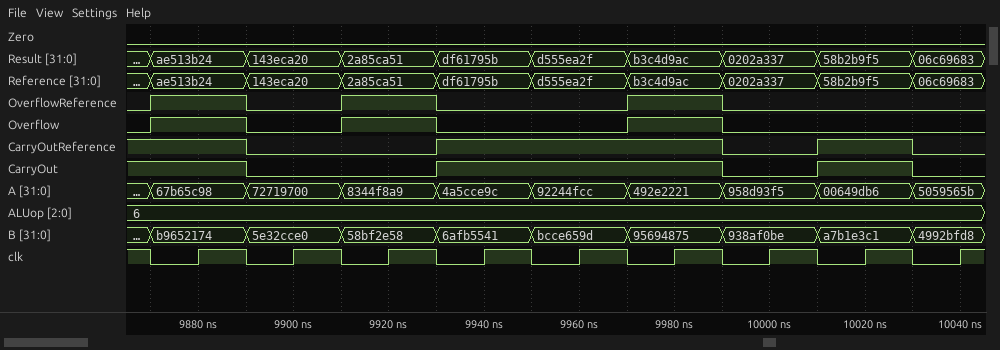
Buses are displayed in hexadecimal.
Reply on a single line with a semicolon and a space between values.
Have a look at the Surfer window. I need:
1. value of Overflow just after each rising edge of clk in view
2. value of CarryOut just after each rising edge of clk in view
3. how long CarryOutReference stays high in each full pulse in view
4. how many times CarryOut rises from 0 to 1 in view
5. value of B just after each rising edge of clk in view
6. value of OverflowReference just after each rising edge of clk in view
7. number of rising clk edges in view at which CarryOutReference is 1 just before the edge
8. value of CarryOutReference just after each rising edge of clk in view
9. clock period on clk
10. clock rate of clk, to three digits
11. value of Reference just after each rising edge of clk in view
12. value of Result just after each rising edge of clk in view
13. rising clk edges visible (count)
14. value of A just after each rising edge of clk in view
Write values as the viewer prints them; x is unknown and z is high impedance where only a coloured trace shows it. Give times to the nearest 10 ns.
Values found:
1 0 1 0 0 1 0 0 0; 1 0 0 1 1 1 0 1 0; 60 ns, 20 ns; 2; b9652174, 5e32cce0, 58bf2e58, 6afb5541, bcce659d, 95694875, 938af0be, a7b1e3c1, 4992bfd8; 1 0 1 0 0 1 0 0 0; 5; 1 0 0 1 1 1 0 1 0; 20 ns; 50.0 MHz; ae513b24, 143eca20, 2a85ca51, df61795b, d555ea2f, b3c4d9ac, 0202a337, 58b2b9f5, 06c69683; ae513b24, 143eca20, 2a85ca51, df61795b, d555ea2f, b3c4d9ac, 0202a337, 58b2b9f5, 06c69683; 9; 67b65c98, 72719700, 8344f8a9, 4a5cce9c, 92244fcc, 492e2221, 958d93f5, 00649db6, 5059565b
